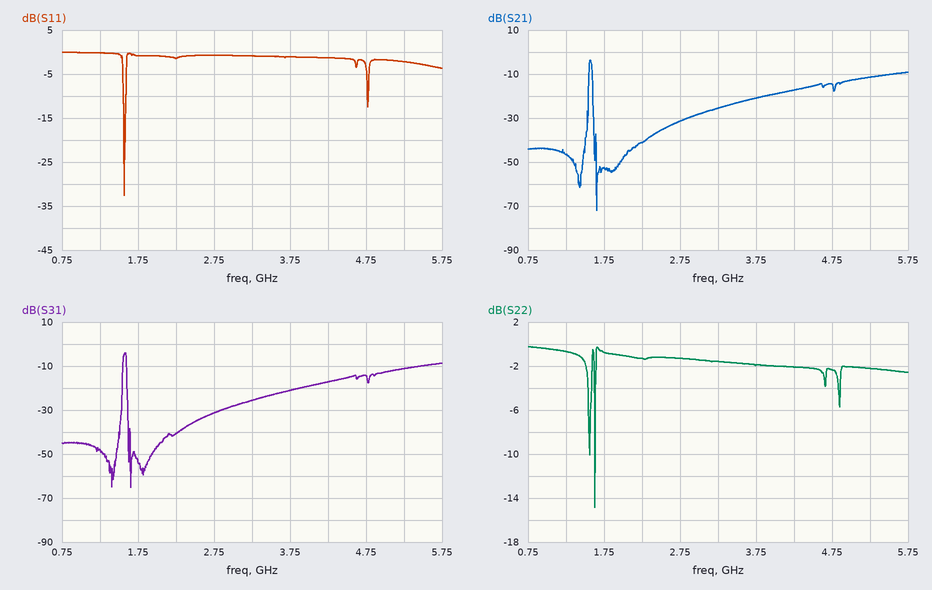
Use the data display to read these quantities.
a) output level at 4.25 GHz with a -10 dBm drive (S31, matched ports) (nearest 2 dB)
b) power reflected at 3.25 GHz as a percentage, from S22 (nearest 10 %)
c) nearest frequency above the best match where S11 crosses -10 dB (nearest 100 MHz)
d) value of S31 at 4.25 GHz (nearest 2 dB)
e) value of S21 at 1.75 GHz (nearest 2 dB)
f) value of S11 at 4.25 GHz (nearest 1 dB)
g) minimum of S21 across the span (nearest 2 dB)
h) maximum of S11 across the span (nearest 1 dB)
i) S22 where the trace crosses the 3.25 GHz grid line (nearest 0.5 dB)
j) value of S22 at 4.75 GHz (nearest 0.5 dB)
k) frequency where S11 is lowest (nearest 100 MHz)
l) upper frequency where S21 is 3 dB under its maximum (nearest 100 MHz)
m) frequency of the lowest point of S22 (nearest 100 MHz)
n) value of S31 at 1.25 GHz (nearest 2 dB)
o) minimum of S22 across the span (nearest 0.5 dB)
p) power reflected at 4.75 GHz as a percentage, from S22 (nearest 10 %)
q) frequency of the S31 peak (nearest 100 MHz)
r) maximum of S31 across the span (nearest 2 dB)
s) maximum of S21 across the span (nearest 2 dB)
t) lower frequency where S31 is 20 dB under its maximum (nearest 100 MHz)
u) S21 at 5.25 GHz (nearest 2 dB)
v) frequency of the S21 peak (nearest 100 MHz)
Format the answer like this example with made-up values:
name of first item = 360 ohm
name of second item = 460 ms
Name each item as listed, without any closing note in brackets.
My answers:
output level at 4.25 GHz with a -10 dBm drive (S31, matched ports) = -28 dBm
power reflected at 3.25 GHz as a percentage, from S22 = 70 %
nearest frequency above the best match where S11 crosses -10 dB = 1.6 GHz
value of S31 at 4.25 GHz = -18 dB
value of S21 at 1.75 GHz = -52 dB
value of S11 at 4.25 GHz = -1 dB
minimum of S21 across the span = -72 dB
maximum of S11 across the span = 0 dB
S22 where the trace crosses the 3.25 GHz grid line = -1.5 dB
value of S22 at 4.75 GHz = -2.5 dB
frequency where S11 is lowest = 1.6 GHz
upper frequency where S21 is 3 dB under its maximum = 1.6 GHz
frequency of the lowest point of S22 = 1.6 GHz
value of S31 at 1.25 GHz = -48 dB
minimum of S22 across the span = -15.0 dB
power reflected at 4.75 GHz as a percentage, from S22 = 60 %
frequency of the S31 peak = 1.6 GHz
maximum of S31 across the span = -4 dB
maximum of S21 across the span = -4 dB
lower frequency where S31 is 20 dB under its maximum = 1.5 GHz
S21 at 5.25 GHz = -12 dB
frequency of the S21 peak = 1.6 GHz
